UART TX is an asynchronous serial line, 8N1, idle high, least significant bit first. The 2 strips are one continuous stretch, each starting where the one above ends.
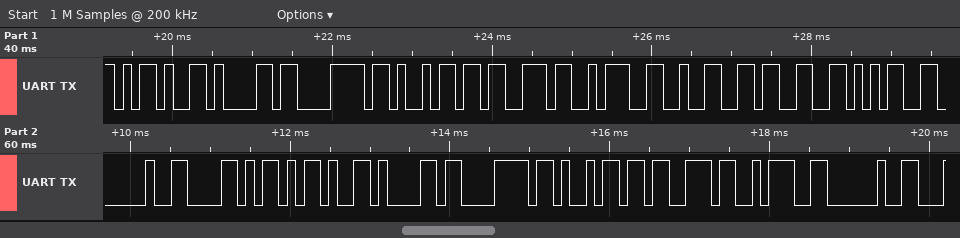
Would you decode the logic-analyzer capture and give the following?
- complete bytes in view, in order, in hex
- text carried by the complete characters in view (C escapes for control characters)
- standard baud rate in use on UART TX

2D 61 78 69 73 3A 32 33 35 20 58 2D 61 78 69 73 3A 20
"-axis:235 X-axis: "
9600 baud
